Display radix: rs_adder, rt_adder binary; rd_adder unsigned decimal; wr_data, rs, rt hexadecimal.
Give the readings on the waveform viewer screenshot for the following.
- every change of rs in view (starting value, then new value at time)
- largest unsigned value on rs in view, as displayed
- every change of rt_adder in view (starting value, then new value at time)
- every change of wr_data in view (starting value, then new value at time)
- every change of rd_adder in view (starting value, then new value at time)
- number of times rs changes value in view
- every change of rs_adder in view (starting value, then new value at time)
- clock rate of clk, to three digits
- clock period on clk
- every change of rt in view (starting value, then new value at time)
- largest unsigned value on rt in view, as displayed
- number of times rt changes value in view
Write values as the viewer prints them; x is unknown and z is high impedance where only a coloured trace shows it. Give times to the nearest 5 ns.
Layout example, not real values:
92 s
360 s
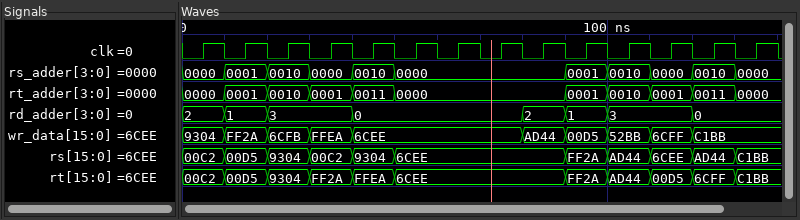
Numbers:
00C2, 00D5 at 10 ns, 9304 at 20 ns, 00C2 at 30 ns, 9304 at 40 ns, 6CEE at 50 ns, FF2A at 90 ns, AD44 at 100 ns, 6CEE at 110 ns, AD44 at 120 ns, C1BB at 130 ns
FF2A
0000, 0001 at 10 ns, 0010 at 20 ns, 0001 at 30 ns, 0011 at 40 ns, 0000 at 50 ns, 0001 at 90 ns, 0010 at 100 ns, 0001 at 110 ns, 0011 at 120 ns, 0000 at 130 ns
9304, FF2A at 10 ns, 6CFB at 20 ns, FFEA at 30 ns, 6CEE at 40 ns, AD44 at 80 ns, 00D5 at 90 ns, 52BB at 100 ns, 6CFF at 110 ns, C1BB at 120 ns
2, 1 at 10 ns, 3 at 20 ns, 0 at 40 ns, 2 at 80 ns, 1 at 90 ns, 3 at 100 ns, 0 at 120 ns
10
0000, 0001 at 10 ns, 0010 at 20 ns, 0000 at 30 ns, 0010 at 40 ns, 0000 at 50 ns, 0001 at 90 ns, 0010 at 100 ns, 0000 at 110 ns, 0010 at 120 ns, 0000 at 130 ns
100 MHz
10 ns
00C2, 00D5 at 10 ns, 9304 at 20 ns, FF2A at 30 ns, FFEA at 40 ns, 6CEE at 50 ns, FF2A at 90 ns, AD44 at 100 ns, 00D5 at 110 ns, 6CFF at 120 ns, C1BB at 130 ns
FFEA
10
